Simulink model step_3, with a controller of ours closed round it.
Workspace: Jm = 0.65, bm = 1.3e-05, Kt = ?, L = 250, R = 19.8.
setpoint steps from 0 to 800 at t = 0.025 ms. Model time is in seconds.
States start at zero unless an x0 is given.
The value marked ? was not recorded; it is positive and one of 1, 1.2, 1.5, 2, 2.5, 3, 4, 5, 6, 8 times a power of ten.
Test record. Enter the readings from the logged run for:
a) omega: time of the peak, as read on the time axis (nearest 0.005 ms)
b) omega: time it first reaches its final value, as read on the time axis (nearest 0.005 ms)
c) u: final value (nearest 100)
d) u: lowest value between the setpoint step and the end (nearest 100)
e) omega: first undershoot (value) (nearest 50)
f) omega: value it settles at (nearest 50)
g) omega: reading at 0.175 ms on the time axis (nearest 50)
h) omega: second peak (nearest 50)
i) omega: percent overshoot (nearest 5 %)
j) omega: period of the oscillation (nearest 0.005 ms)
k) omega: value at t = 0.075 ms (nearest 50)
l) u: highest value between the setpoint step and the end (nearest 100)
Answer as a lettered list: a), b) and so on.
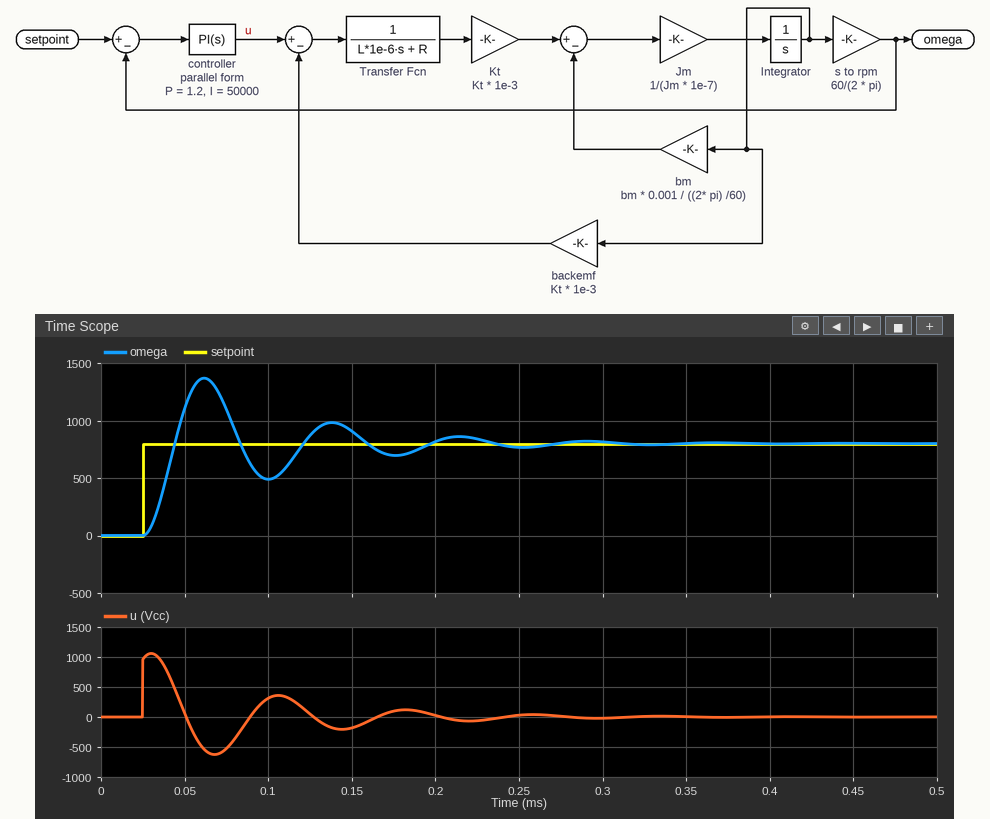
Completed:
a) 0.060 ms
b) 0.045 ms
c) 0
d) -600
e) 500
f) 800
g) 700
h) 1000
i) 70 %
j) 0.075 ms
k) 1100
l) 1100
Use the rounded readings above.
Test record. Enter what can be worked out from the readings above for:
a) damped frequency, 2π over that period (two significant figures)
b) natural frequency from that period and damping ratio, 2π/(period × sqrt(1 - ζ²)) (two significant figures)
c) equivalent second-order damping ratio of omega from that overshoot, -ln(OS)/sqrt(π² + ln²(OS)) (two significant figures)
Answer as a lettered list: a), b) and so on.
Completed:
a) 84 rad/ms
b) 84 rad/ms
c) 0.11
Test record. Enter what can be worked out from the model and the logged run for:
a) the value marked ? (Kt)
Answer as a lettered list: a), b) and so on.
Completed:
a) 12
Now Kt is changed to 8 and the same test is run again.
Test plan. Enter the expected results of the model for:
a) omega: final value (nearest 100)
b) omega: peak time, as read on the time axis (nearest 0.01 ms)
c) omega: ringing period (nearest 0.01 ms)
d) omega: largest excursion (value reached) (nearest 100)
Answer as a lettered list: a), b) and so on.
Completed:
a) 800
b) 0.07 ms
c) 0.10 ms
d) 1400
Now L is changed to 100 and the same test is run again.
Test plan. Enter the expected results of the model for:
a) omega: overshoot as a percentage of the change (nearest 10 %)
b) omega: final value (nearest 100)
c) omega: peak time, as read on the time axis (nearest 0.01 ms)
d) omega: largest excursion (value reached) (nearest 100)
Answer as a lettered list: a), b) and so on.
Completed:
a) 40 %
b) 800
c) 0.05 ms
d) 1100
